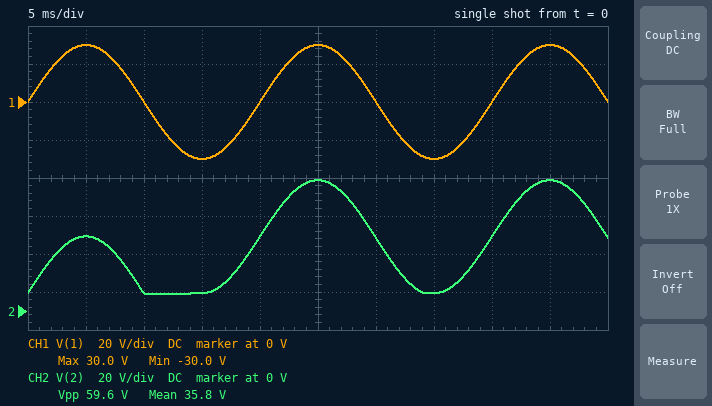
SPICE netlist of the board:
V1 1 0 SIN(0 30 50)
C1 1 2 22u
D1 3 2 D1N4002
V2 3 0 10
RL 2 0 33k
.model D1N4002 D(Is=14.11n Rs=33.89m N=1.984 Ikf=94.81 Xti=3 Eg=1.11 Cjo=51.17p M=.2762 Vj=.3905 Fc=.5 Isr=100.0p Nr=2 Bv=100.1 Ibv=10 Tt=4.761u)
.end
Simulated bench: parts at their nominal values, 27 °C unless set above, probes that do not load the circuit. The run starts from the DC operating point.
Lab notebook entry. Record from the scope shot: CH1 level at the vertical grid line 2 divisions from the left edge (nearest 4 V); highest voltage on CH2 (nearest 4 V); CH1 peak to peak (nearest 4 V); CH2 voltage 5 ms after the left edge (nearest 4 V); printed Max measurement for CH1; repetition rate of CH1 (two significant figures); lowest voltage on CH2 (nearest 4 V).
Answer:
0 V
68 V
60 V
40 V
30.0 V
50 Hz
8 V
